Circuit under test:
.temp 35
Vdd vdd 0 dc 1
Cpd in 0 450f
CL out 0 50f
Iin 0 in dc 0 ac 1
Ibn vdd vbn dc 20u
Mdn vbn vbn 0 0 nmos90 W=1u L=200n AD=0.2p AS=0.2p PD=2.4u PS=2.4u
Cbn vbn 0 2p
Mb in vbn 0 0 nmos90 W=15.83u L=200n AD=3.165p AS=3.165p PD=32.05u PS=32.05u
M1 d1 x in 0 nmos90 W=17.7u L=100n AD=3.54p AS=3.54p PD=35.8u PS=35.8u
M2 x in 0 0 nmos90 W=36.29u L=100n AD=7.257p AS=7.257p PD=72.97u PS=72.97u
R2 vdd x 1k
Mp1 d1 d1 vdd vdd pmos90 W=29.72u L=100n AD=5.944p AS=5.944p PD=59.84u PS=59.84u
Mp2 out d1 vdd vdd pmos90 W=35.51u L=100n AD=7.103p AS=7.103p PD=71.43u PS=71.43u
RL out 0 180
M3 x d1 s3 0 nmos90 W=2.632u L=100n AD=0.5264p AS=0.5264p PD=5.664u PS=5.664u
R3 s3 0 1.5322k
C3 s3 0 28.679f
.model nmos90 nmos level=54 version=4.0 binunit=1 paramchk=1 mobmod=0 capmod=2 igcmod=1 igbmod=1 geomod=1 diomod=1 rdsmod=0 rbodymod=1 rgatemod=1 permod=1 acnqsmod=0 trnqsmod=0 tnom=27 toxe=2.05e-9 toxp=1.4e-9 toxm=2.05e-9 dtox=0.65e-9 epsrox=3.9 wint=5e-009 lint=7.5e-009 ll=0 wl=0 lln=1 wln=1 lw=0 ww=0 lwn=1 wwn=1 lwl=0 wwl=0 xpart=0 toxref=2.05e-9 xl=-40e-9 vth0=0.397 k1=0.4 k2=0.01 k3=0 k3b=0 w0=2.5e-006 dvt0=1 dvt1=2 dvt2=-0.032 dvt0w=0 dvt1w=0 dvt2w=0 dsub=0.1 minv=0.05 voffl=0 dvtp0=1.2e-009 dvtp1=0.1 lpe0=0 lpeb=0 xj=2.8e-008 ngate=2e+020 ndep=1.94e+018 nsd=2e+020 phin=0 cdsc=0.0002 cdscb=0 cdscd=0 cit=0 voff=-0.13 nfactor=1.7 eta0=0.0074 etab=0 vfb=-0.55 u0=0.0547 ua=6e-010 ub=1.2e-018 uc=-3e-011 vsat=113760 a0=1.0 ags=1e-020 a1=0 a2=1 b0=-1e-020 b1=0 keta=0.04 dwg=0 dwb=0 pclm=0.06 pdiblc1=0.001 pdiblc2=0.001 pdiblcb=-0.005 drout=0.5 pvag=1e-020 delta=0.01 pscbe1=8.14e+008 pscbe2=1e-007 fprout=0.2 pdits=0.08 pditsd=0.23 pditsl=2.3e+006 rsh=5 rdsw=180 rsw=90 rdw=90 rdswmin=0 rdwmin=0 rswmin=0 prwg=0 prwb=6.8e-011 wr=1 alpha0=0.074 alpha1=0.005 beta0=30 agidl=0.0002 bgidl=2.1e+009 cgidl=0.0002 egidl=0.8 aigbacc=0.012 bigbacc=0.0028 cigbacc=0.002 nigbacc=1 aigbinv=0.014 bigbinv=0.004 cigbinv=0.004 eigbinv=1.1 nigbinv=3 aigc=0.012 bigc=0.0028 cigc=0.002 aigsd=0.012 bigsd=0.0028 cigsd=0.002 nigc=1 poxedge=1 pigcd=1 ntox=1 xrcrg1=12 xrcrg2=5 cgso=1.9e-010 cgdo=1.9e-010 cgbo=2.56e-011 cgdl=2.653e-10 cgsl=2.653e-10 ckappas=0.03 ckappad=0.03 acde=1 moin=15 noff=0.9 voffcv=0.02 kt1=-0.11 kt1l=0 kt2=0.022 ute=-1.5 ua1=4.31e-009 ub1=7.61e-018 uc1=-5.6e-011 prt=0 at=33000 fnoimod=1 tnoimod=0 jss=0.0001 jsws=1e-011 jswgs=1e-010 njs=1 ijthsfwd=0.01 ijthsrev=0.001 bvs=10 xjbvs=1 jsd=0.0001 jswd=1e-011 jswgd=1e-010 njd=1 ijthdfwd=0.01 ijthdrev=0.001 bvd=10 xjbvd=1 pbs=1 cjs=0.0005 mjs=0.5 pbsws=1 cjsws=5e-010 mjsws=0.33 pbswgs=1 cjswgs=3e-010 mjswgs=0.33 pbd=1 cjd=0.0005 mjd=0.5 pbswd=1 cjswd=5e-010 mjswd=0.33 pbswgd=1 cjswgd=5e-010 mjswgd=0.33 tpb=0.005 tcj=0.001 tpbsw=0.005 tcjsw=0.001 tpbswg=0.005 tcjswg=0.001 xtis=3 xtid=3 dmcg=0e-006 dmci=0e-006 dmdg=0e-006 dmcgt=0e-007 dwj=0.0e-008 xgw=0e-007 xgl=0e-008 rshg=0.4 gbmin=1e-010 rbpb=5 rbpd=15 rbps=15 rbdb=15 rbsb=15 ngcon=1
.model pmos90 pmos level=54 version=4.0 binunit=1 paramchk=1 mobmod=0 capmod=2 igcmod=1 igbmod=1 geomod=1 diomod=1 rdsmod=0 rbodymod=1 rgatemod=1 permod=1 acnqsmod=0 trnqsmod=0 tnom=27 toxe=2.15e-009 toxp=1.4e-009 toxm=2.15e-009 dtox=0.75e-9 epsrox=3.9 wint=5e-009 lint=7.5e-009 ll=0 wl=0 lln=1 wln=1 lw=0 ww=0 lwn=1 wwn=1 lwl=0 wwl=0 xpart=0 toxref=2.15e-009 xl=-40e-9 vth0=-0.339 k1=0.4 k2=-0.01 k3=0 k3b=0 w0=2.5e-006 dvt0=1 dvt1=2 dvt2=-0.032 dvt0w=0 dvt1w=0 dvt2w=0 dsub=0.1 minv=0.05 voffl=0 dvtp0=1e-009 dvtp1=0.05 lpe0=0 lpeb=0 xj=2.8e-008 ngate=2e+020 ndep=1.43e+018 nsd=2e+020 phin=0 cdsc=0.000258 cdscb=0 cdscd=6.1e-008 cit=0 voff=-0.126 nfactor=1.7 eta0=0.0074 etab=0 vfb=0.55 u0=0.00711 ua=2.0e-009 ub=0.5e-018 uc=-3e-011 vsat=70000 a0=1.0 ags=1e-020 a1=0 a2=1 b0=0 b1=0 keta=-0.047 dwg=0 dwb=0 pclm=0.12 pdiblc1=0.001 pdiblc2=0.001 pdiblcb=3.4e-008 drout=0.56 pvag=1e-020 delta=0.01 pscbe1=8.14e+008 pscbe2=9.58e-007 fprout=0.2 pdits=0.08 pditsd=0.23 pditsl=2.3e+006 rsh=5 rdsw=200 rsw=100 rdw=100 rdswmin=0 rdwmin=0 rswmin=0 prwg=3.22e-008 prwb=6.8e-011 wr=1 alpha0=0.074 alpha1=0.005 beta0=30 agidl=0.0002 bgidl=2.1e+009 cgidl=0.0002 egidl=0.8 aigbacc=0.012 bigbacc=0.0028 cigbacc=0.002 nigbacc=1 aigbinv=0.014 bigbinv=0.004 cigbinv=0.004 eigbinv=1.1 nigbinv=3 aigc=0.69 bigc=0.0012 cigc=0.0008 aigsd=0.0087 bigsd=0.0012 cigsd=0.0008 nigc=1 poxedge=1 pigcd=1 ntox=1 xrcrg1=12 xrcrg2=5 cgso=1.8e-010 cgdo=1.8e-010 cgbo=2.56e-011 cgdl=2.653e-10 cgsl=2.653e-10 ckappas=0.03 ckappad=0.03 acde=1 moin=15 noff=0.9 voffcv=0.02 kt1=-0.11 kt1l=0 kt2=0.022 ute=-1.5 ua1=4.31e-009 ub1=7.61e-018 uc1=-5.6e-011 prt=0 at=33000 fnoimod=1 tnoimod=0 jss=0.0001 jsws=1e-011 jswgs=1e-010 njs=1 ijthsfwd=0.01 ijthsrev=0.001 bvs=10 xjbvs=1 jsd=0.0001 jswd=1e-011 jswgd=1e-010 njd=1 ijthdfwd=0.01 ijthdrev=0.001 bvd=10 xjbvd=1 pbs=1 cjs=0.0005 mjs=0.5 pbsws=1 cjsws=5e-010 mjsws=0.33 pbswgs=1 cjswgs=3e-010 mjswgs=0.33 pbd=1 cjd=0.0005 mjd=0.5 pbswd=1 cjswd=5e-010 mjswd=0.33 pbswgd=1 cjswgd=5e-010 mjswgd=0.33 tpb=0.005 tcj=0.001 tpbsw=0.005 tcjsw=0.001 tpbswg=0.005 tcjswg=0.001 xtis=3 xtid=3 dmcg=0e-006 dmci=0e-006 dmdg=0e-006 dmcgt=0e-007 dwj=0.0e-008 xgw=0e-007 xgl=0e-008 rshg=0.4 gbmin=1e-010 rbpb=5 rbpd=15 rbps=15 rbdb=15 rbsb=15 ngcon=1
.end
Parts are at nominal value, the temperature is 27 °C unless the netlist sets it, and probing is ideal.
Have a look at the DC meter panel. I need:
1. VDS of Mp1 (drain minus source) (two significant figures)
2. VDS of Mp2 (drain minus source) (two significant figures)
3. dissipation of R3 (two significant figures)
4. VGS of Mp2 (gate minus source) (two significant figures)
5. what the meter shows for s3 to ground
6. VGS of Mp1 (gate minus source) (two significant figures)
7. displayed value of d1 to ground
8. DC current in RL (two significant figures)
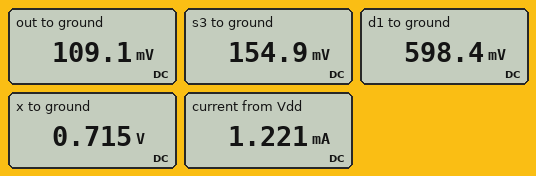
-400 mV
-890 mV
16 µW
-400 mV
154.9 mV
-400 mV
598.4 mV
610 µA
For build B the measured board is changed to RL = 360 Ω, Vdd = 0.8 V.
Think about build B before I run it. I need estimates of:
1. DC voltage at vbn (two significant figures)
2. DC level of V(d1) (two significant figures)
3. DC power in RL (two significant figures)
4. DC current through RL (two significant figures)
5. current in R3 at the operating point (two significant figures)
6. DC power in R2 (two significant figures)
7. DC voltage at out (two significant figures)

460 mV
400 mV
79 µW
470 µA
34 µA
14 µW
170 mV
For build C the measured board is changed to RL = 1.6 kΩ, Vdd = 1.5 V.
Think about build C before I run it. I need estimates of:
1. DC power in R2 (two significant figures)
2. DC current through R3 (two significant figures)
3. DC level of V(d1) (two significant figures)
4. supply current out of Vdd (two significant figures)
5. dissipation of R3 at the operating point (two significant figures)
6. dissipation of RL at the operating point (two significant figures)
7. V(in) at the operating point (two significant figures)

570 µW
300 µA
1.1 V
1.6 mA
140 µW
410 µW
330 mV
